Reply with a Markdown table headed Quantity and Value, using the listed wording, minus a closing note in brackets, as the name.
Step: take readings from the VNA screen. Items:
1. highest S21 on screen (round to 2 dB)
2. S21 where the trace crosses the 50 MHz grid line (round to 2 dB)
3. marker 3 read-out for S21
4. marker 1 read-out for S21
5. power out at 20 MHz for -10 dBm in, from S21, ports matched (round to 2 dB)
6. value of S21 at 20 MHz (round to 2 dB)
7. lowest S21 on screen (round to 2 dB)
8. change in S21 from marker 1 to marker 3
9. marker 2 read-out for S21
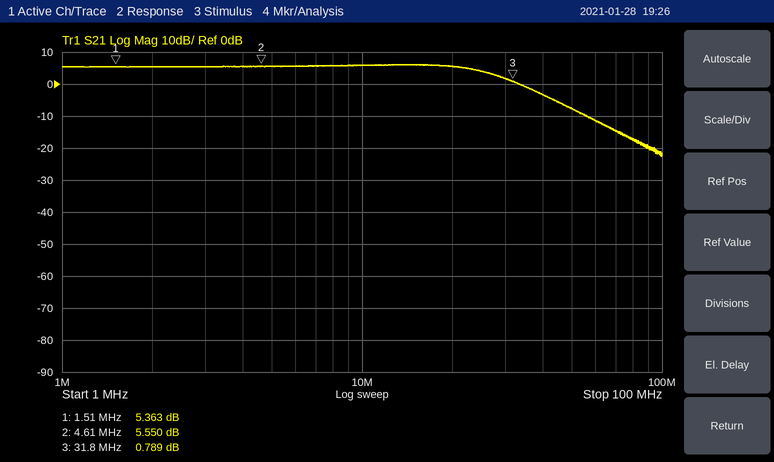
| Quantity | Value |
|---|---|
| highest S21 on screen | 6 dB |
| S21 where the trace crosses the 50 MHz grid line | -8 dB |
| marker 3 read-out for S21 | 0.789 dB |
| marker 1 read-out for S21 | 5.363 dB |
| power out at 20 MHz for -10 dBm in, from S21, ports matched | -4 dBm |
| value of S21 at 20 MHz | 6 dB |
| lowest S21 on screen | -22 dB |
| change in S21 from marker 1 to marker 3 | -4.574 dB |
| marker 2 read-out for S21 | 5.550 dB |
